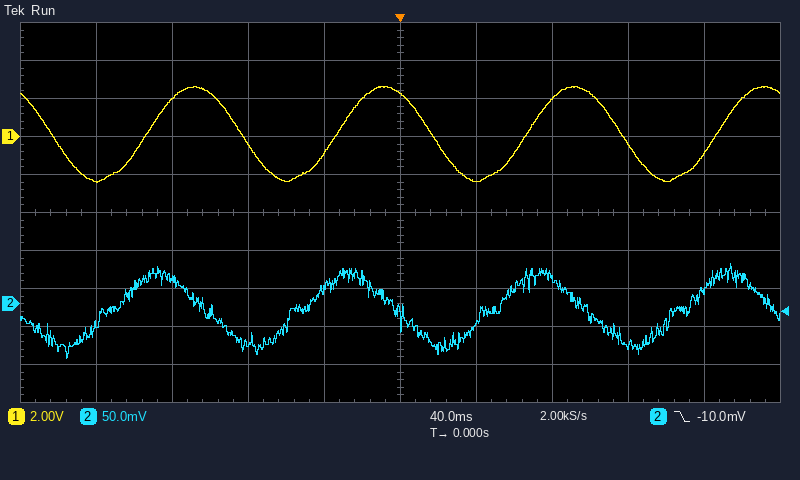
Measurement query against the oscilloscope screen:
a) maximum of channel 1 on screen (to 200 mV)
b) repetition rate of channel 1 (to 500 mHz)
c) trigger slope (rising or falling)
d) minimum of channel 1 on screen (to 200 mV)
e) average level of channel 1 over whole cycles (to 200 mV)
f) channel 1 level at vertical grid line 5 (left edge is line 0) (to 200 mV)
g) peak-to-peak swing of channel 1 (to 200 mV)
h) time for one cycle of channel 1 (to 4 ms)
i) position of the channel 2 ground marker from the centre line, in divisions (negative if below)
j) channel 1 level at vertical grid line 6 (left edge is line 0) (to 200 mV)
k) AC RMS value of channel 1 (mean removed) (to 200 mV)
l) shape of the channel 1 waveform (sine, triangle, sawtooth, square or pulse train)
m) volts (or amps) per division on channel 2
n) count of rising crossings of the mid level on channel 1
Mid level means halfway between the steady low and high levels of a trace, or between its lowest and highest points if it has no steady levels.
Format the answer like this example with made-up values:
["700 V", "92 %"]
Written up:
["2.6 V", "10.0 Hz", "falling", "-2.4 V", "200 mV", "2.2 V", "5.0 V", "100 ms", "-2.4 div", "-2.4 V", "1.8 V", "sine", "50 mV", "4"]
